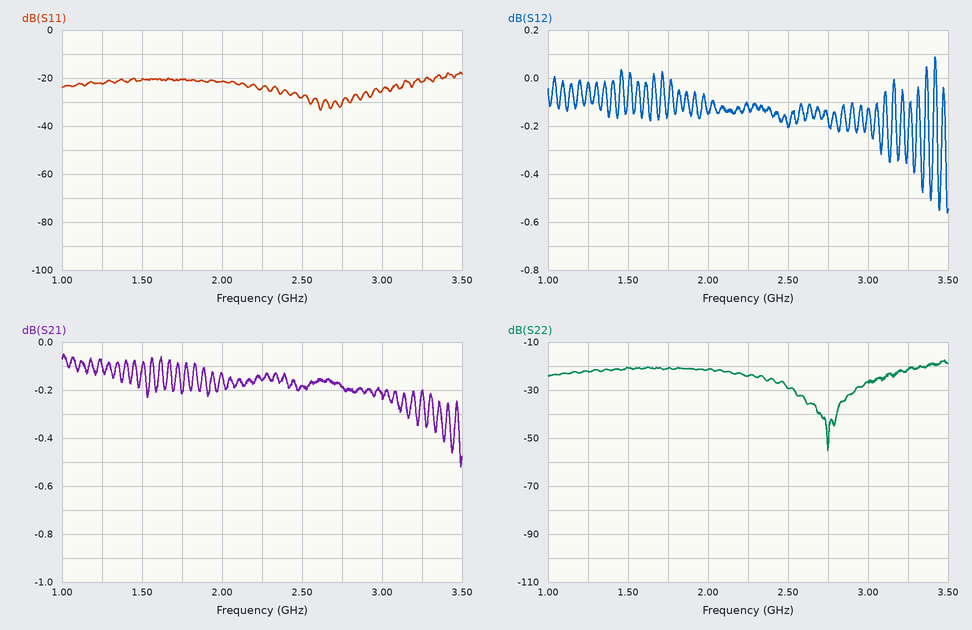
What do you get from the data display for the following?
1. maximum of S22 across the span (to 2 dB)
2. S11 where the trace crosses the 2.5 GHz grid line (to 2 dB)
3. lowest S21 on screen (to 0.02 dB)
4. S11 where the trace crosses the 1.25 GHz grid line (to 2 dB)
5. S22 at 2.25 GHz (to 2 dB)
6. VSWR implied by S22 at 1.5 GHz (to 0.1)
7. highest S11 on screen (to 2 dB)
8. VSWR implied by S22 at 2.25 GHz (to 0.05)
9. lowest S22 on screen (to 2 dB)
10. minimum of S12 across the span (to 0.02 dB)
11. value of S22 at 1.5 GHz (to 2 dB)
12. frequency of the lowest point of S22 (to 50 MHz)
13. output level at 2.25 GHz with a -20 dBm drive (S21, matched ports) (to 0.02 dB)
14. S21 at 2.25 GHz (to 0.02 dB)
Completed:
-18 dB
-28 dB
-0.52 dB
-22 dB
-24 dB
1.2
-18 dB
1.15
-56 dB
-0.56 dB
-20 dB
2.75 GHz
-20.16 dBm
-0.16 dB
